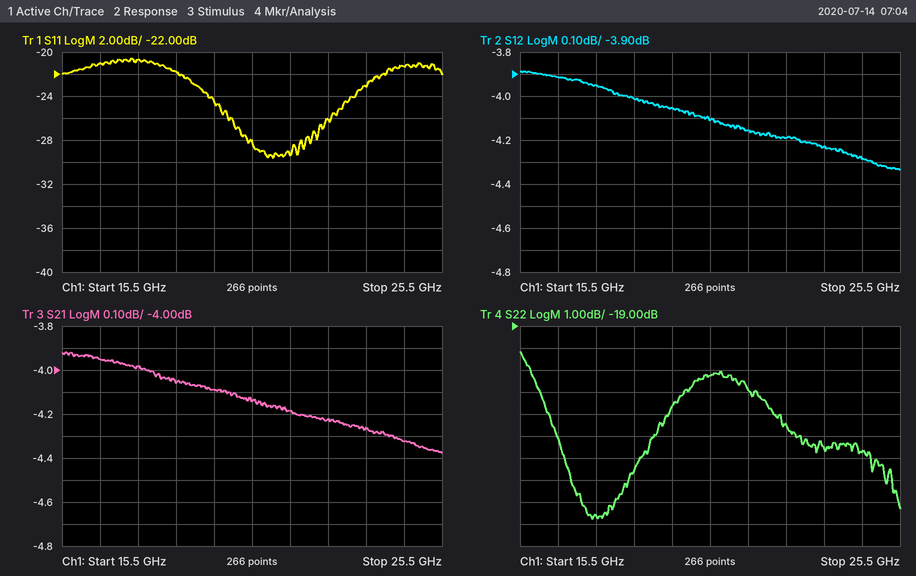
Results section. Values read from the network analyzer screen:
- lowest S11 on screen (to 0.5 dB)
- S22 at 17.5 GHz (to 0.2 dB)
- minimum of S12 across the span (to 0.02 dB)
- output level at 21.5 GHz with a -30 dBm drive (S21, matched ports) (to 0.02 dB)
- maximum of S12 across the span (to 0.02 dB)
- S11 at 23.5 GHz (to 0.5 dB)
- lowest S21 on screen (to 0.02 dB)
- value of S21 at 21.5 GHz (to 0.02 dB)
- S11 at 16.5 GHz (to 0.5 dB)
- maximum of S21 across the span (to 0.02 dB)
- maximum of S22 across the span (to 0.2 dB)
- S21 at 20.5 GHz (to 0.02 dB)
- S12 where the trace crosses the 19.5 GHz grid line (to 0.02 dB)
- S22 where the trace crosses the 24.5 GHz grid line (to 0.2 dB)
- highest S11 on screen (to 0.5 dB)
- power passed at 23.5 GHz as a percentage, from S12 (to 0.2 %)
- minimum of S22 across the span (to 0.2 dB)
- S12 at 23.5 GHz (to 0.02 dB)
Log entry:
-29.5 dB
-27.6 dB
-4.34 dB
-34.18 dBm
-3.88 dB
-23.0 dB
-4.38 dB
-4.18 dB
-21.0 dB
-3.92 dB
-20.2 dB
-4.14 dB
-4.06 dB
-24.8 dB
-20.5 dB
37.8 %
-27.8 dB
-4.22 dB
